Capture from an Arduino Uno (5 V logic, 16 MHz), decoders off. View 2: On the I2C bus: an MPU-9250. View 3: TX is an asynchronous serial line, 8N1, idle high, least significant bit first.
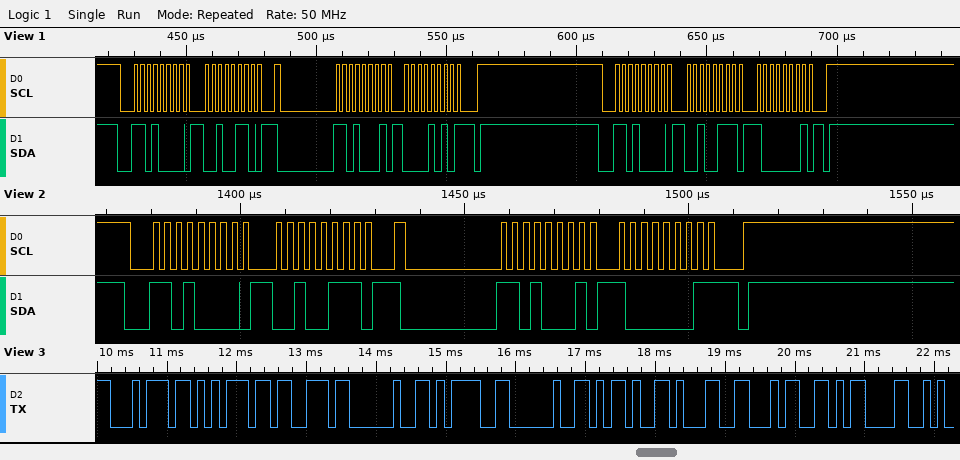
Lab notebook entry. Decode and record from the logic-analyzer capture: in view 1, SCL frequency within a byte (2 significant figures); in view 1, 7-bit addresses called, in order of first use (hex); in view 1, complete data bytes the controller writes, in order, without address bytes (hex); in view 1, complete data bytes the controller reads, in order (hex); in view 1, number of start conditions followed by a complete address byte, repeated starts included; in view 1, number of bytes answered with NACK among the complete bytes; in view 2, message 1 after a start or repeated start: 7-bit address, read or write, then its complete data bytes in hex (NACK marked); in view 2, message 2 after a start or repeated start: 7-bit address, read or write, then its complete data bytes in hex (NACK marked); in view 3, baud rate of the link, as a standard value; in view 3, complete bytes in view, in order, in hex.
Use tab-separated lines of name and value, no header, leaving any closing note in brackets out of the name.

in view 1, SCL frequency within a byte	400 kHz
in view 1, 7-bit addresses called, in order of first use	0x68
in view 1, complete data bytes the controller writes, in order, without address bytes	26 27 81
in view 1, complete data bytes the controller reads, in order	0A
in view 1, number of start conditions followed by a complete address byte, repeated starts included	3
in view 1, number of bytes answered with NACK among the complete bytes	1
in view 2, message 1 after a start or repeated start: 7-bit address, read or write, then its complete data bytes in hex	0x68 write: 27
in view 2, message 2 after a start or repeated start: 7-bit address, read or write, then its complete data bytes in hex	0x68 read: 81 NACK
in view 3, baud rate of the link, as a standard value	9600 baud
in view 3, complete bytes in view, in order, in hex	74 75 73 20 3D 20 2D 31 34 0D
